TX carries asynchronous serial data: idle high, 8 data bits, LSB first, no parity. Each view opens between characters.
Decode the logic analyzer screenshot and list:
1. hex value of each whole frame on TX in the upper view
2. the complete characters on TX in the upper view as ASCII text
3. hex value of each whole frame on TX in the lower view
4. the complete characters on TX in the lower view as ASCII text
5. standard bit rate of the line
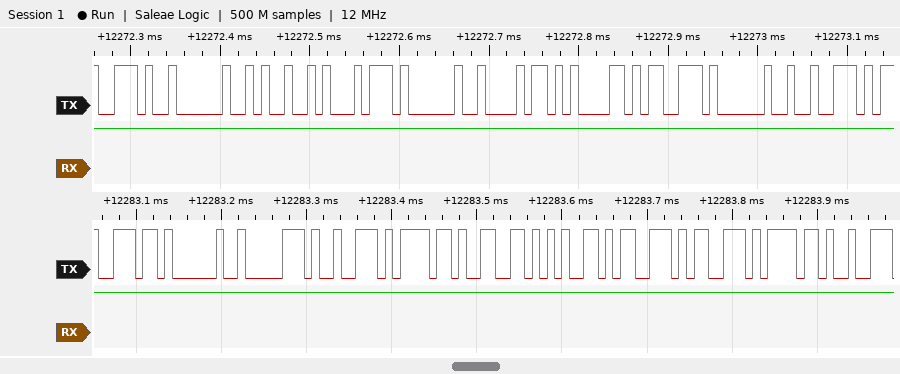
2E, 20, 49, 74, 20, 68, 61, 73, 20, 72
". It has r"
6E, 20, 70, 72, 6F, 66, 65, 73, 73, 6F
"n professo"
115200 baud
